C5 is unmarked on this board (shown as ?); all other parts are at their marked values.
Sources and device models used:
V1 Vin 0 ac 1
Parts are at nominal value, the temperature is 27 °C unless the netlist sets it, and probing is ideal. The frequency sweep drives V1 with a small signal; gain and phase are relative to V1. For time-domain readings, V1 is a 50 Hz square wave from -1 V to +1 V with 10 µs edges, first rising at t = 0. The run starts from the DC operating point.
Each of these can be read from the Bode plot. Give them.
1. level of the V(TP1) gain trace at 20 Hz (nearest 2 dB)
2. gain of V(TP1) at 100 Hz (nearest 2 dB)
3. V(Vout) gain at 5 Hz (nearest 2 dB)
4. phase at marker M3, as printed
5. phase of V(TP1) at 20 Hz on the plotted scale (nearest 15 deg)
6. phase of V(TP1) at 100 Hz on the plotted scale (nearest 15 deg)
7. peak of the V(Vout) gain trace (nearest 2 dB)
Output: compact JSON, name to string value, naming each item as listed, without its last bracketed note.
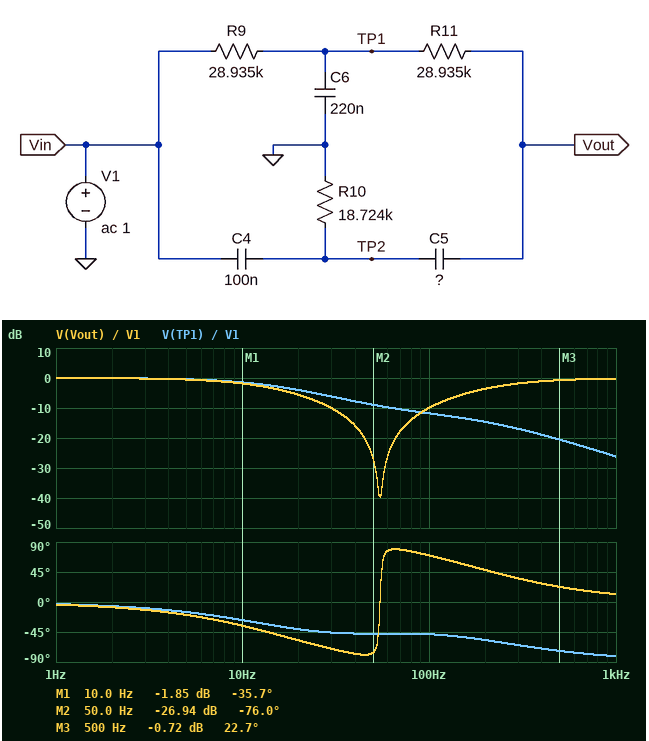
{"level of the V(TP1) gain trace at 20 Hz": "-4 dB", "gain of V(TP1) at 100 Hz": "-12 dB", "V(Vout) gain at 5 Hz": "0 dB", "phase at marker M3, as printed": "22.7 deg", "phase of V(TP1) at 20 Hz on the plotted scale": "-45 deg", "phase of V(TP1) at 100 Hz on the plotted scale": "-45 deg", "peak of the V(Vout) gain trace": "0 dB"}
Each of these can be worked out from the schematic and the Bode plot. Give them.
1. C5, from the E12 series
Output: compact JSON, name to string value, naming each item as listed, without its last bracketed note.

{"C5, from the E12 series": "82 nF"}
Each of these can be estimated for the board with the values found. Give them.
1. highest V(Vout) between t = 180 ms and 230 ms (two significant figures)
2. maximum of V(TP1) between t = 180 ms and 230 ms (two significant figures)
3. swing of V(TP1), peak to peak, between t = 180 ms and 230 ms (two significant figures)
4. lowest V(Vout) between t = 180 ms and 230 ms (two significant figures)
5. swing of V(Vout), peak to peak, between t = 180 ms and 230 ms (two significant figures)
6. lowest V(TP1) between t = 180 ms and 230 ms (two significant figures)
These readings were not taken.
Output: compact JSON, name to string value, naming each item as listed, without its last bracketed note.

{"highest V(Vout) between t = 180 ms and 230 ms": "1.6 V", "maximum of V(TP1) between t = 180 ms and 230 ms": "540 mV", "swing of V(TP1), peak to peak, between t = 180 ms and 230 ms": "1.1 V", "lowest V(Vout) between t = 180 ms and 230 ms": "-1.6 V", "swing of V(Vout), peak to peak, between t = 180 ms and 230 ms": "3.3 V", "lowest V(TP1) between t = 180 ms and 230 ms": "-540 mV"}
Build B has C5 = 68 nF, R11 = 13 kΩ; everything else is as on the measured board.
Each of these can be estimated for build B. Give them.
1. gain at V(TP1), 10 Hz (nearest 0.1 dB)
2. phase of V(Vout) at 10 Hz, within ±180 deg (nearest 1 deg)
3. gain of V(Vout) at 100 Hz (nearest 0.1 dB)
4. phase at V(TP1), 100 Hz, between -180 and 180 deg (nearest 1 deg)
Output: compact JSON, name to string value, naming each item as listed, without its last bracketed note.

{"gain at V(TP1), 10 Hz": "-1.3 dB", "phase of V(Vout) at 10 Hz, within ±180 deg": "-30 deg", "gain of V(Vout) at 100 Hz": "-19.7 dB", "phase at V(TP1), 100 Hz, between -180 and 180 deg": "-42 deg"}
